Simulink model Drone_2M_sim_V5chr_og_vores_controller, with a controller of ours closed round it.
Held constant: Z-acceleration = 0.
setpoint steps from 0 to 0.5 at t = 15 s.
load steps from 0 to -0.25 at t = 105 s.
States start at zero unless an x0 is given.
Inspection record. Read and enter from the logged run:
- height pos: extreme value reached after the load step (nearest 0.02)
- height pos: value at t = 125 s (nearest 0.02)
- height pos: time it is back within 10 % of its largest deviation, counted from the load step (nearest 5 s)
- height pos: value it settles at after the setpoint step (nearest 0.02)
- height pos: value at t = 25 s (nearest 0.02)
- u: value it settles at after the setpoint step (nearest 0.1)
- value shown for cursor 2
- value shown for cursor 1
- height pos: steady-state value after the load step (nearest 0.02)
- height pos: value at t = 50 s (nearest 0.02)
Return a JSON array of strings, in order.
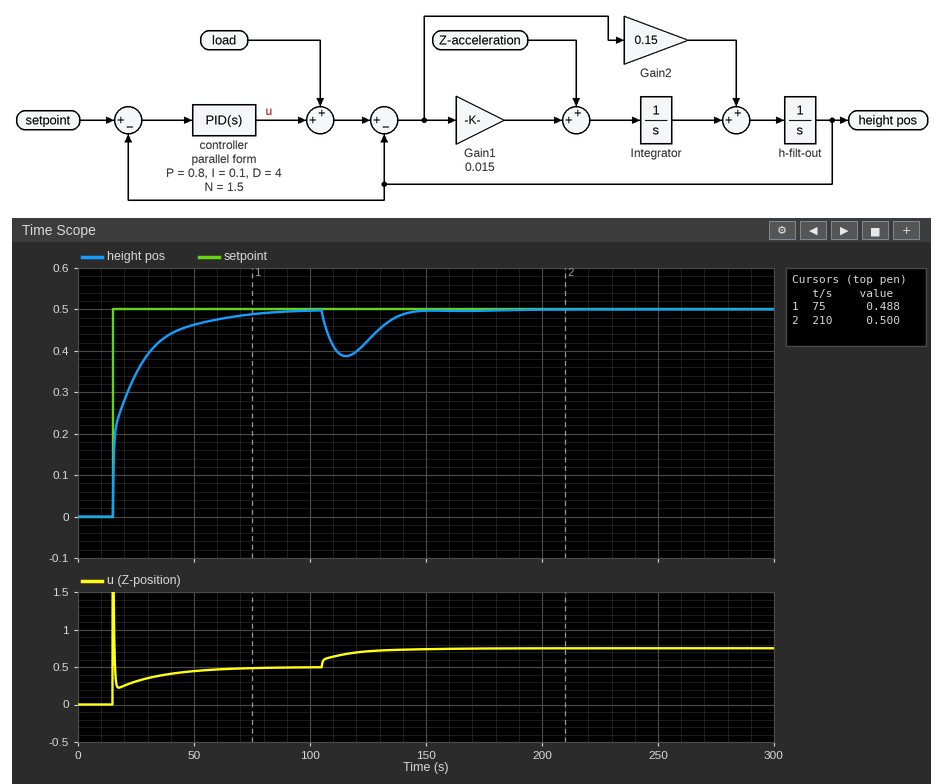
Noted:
["0.38", "0.42", "35 s", "0.50", "0.34", "0.5", "0.500", "0.488", "0.50", "0.46"]
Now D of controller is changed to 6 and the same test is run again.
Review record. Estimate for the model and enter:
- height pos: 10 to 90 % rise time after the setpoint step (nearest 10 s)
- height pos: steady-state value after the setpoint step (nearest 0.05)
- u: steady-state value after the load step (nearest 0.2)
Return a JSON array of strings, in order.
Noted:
["30 s", "0.50", "0.8"]
